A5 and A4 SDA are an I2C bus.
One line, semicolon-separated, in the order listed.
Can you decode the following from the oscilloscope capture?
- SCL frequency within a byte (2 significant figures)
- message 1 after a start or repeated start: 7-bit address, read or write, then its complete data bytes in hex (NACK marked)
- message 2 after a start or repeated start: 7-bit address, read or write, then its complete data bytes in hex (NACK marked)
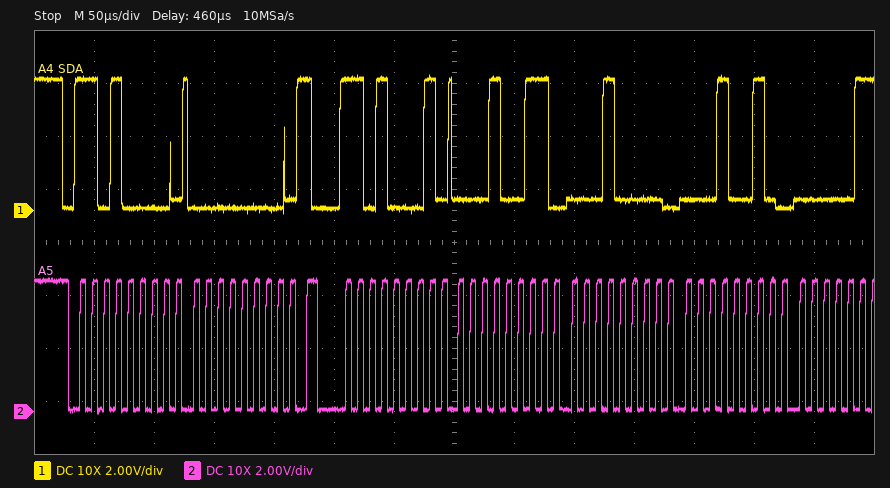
100 kHz; 0x68 write: 00; 0x68 read: 13 10 12
